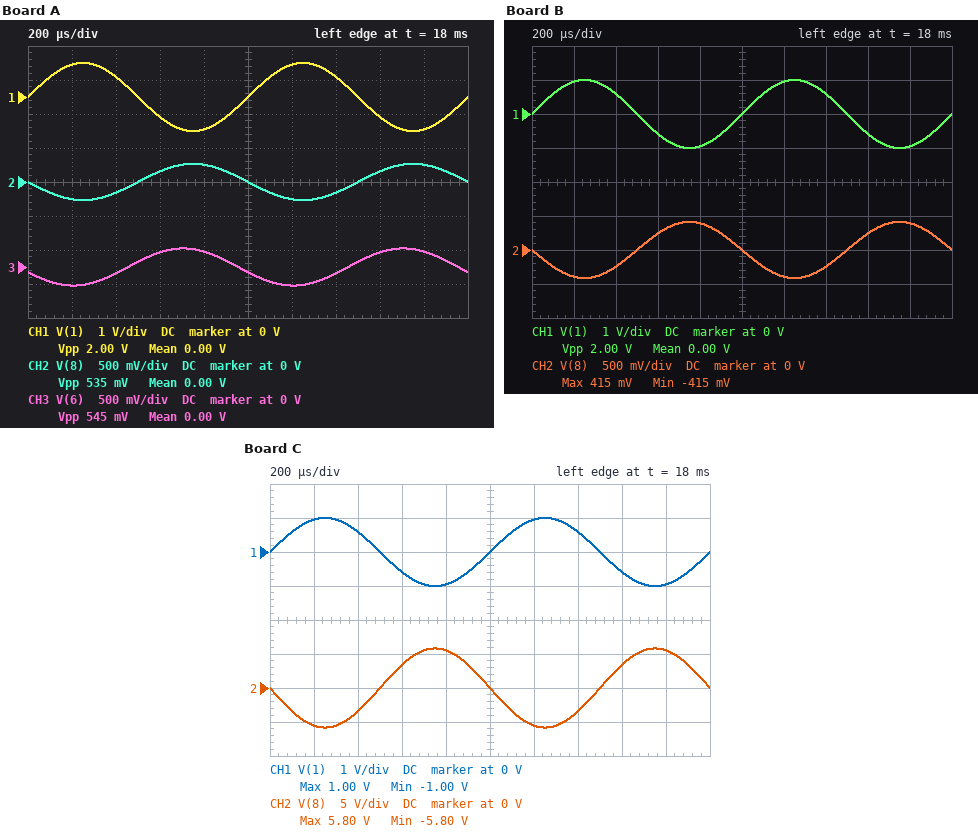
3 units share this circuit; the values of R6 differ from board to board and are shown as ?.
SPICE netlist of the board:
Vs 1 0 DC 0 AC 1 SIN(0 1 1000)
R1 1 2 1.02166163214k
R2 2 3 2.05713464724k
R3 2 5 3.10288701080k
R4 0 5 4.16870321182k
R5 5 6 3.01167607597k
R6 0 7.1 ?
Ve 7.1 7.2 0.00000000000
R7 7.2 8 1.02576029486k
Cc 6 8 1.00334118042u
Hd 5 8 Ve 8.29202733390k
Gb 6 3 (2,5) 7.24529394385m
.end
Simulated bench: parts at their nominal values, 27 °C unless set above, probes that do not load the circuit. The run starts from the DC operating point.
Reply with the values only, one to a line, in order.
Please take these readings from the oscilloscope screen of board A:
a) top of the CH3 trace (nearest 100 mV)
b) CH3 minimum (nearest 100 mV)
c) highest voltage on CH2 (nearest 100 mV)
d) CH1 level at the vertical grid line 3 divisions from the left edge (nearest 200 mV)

300 mV
-300 mV
300 mV
-600 mV
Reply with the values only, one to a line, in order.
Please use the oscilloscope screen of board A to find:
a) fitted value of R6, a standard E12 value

820 Ω
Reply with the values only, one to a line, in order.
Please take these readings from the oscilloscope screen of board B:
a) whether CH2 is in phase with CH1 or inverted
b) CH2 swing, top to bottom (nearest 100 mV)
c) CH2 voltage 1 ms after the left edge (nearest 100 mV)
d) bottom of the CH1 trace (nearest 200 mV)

inverted
800 mV
0 V
-1.0 V
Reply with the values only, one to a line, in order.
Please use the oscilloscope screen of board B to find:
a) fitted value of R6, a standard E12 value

1.5 kΩ
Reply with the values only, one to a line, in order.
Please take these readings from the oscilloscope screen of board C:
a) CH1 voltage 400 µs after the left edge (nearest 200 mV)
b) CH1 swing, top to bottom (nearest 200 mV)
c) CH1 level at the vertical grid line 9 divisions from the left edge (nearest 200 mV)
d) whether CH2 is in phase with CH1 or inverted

600 mV
2.0 V
-1.0 V
inverted
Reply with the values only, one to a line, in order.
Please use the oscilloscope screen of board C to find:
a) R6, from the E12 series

5.6 kΩ
